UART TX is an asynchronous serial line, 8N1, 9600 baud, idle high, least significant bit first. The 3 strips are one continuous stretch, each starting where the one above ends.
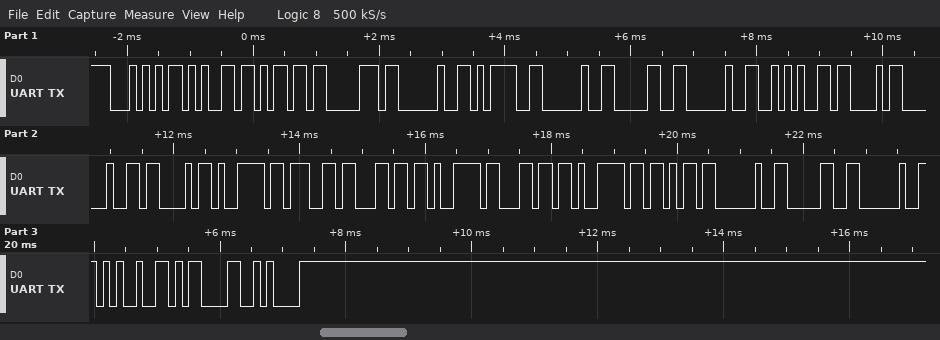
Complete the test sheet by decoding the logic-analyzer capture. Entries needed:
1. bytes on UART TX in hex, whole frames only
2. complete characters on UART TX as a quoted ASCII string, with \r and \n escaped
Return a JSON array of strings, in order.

["54 65 6D 70 20 3D 20 30 20 2A 43 20 43 79 67 6C 79 6C 79 6B 20 30 20 25 0D 0A", "\"Temp = 0 *C Cyglylyk 0 %\\r\\n\""]
